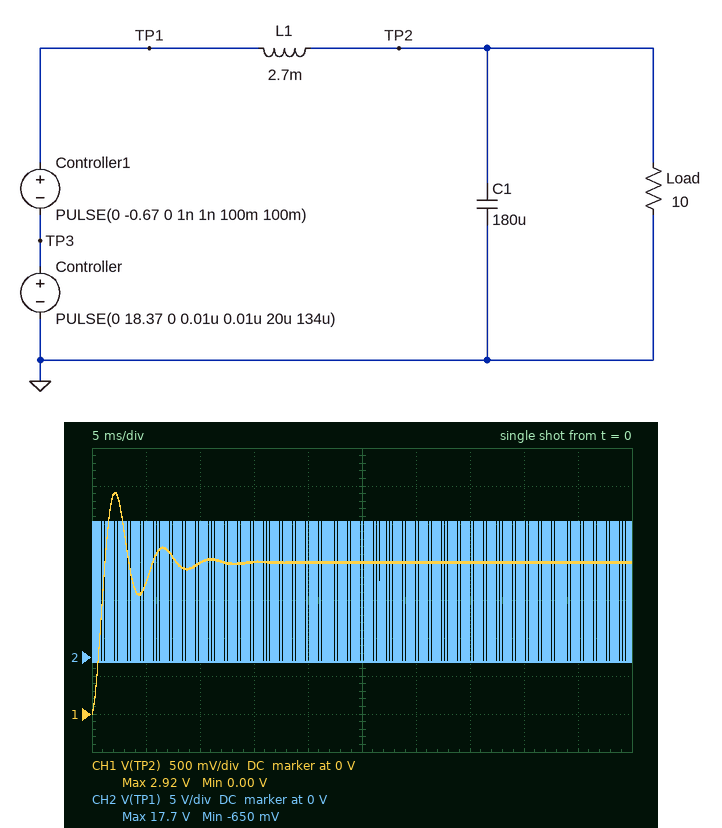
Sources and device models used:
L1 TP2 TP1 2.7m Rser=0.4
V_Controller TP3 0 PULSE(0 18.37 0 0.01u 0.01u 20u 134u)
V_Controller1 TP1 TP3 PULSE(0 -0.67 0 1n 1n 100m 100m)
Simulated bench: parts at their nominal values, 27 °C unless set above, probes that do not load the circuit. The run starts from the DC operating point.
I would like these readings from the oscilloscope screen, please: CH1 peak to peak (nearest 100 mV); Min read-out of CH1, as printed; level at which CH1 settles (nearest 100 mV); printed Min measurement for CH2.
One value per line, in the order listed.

2.9 V
0.00 V
2.0 V
-650 mV
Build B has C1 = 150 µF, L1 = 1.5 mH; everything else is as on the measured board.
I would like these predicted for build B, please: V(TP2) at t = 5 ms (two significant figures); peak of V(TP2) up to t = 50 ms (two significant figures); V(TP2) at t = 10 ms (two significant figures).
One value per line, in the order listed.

2.1 V
3.0 V
2.0 V
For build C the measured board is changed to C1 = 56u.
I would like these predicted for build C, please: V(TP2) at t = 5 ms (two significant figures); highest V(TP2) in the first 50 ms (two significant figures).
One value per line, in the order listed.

2.0 V
2.6 V
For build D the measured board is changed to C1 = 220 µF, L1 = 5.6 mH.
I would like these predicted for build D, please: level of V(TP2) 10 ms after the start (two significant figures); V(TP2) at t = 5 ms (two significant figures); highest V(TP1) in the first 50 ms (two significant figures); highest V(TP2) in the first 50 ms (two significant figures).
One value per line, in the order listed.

2.1 V
2.3 V
18 V
2.8 V
